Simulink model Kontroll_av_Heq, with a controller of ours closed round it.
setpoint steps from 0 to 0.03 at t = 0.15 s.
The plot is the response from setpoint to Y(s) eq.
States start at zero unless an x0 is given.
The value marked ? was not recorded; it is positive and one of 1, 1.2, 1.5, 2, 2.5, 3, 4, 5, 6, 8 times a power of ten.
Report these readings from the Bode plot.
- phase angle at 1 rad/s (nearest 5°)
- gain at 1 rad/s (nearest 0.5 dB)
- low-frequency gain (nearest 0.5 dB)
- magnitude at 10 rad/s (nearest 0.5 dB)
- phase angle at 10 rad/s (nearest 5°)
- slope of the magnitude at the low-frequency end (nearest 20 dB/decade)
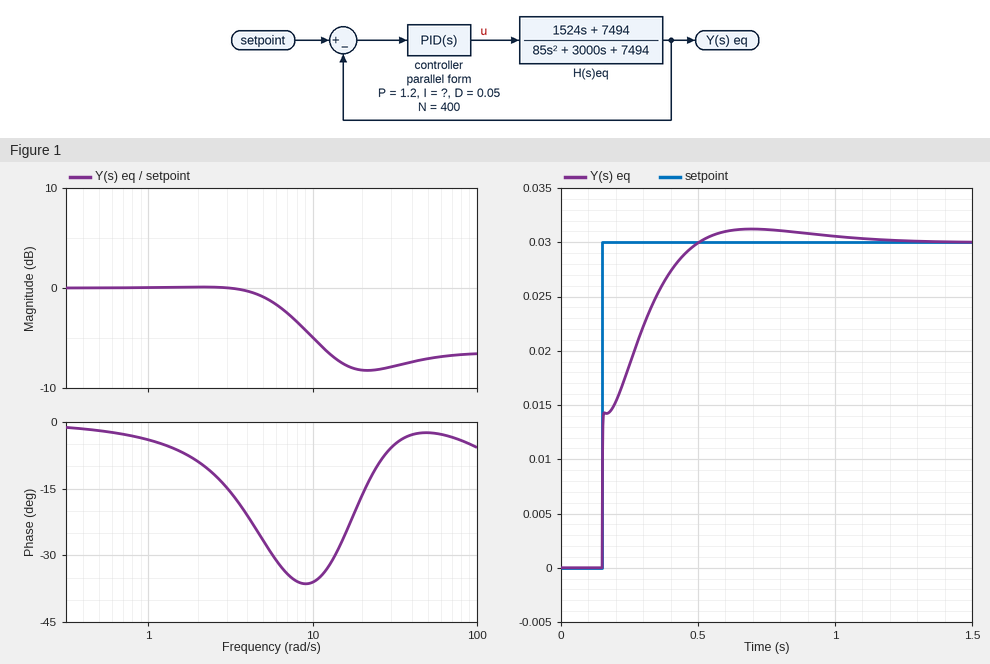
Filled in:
-5°
0.0 dB
0.0 dB
-5.0 dB
-35°
0 dB/decade
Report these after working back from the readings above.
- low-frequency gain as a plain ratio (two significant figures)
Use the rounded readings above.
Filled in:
1.0
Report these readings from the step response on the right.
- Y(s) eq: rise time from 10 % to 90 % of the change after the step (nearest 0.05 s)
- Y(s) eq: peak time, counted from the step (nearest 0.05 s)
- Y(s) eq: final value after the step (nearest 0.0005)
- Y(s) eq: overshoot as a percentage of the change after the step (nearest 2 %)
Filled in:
0.25 s
0.55 s
0.0300
4 %
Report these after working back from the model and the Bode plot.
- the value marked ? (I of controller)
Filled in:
15
